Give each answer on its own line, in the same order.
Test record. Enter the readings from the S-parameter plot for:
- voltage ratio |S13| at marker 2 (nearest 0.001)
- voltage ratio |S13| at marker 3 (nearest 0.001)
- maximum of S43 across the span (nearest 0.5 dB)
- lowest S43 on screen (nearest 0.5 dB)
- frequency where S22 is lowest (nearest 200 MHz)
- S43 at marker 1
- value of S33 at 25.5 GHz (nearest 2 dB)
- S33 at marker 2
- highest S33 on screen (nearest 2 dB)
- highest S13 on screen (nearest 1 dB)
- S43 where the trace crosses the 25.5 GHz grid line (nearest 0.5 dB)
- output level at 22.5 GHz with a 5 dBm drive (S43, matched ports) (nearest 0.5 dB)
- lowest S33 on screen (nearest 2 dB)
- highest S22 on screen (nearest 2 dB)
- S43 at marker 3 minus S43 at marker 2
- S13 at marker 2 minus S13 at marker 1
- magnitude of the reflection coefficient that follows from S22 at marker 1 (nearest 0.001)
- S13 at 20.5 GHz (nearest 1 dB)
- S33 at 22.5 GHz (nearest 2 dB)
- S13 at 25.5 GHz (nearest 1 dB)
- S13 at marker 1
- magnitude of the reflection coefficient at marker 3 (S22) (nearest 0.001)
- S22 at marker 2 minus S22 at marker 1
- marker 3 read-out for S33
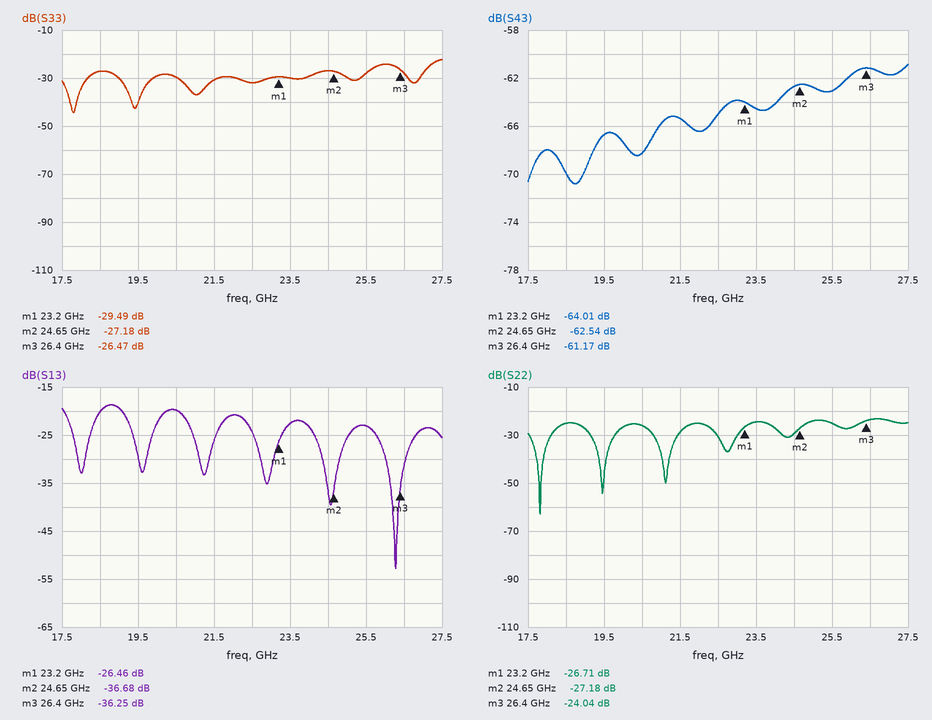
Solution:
0.015
0.015
-61.0 dB
-71.0 dB
17.8 GHz
-64.01 dB
-28 dB
-27.18 dB
-22 dB
-19 dB
-63.0 dB
-60.0 dBm
-44 dB
-24 dB
1.37 dB
-10.22 dB
0.046
-20 dB
-32 dB
-23 dB
-26.46 dB
0.063
-0.47 dB
-26.47 dB
